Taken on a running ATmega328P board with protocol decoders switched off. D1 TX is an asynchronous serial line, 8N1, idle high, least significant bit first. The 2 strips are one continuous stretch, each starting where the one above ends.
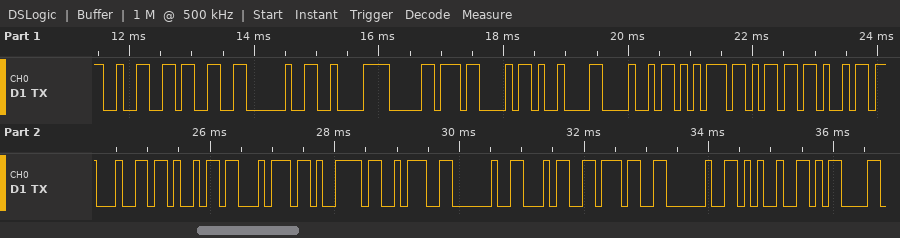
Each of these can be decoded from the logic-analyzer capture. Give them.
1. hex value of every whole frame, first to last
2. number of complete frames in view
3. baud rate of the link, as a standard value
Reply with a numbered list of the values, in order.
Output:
1. 32 33 20 C2 B0 43 09 48 75 6D 69 64 69 74 79 3A 20 34 37 20 25 0D
2. 22
3. 9600 baud
